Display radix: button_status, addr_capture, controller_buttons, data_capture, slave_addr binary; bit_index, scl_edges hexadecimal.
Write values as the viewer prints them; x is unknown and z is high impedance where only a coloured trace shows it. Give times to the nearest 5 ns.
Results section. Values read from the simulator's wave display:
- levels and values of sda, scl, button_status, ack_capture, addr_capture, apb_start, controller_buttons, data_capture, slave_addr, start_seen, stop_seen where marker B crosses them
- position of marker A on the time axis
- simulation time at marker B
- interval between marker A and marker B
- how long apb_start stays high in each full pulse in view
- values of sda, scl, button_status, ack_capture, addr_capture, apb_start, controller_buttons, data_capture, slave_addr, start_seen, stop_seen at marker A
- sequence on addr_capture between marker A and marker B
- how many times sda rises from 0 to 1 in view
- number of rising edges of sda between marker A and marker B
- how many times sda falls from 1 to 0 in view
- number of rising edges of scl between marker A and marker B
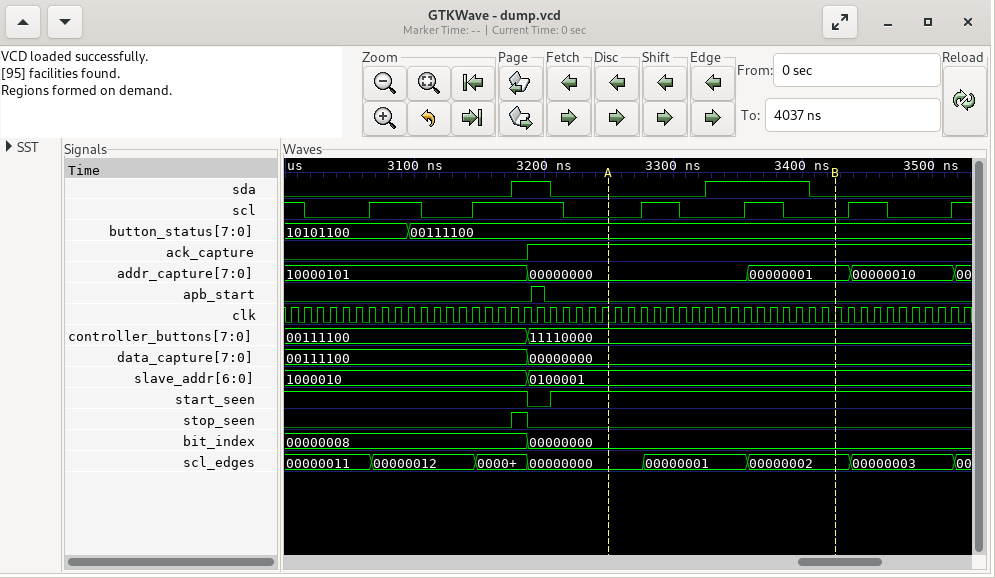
sda=0, scl=0, button_status=00111100, ack_capture=1, addr_capture=00000001, apb_start=0, controller_buttons=11110000, data_capture=00000000, slave_addr=0100001, start_seen=1, stop_seen=0
3250 ns
3425 ns
175 ns
10 ns
sda=0, scl=0, button_status=00111100, ack_capture=1, addr_capture=00000000, apb_start=0, controller_buttons=11110000, data_capture=00000000, slave_addr=0100001, start_seen=1, stop_seen=0
00000000, 00000001
2
1
2
2
